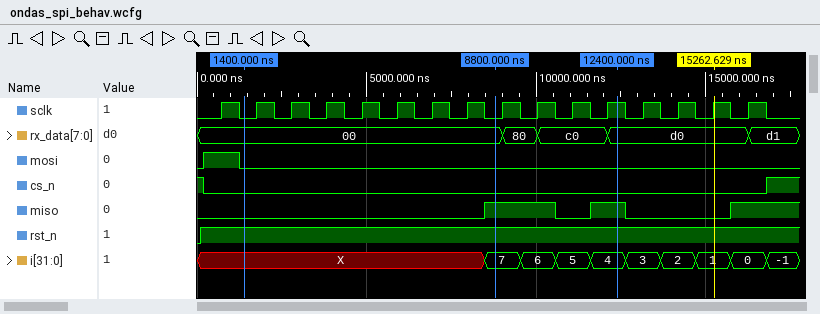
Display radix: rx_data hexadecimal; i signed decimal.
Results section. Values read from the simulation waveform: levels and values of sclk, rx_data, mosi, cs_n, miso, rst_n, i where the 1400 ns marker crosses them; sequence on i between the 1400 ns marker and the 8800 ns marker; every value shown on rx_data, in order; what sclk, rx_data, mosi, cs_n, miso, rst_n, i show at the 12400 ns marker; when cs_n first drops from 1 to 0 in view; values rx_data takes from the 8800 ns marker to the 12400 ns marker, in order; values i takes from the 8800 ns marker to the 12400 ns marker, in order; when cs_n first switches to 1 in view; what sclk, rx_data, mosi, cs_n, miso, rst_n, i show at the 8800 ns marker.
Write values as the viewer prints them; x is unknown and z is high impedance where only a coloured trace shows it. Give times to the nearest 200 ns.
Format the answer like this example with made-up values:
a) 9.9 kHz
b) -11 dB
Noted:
a) sclk=0, rx_data=00, mosi=0, cs_n=0, miso=0, rst_n=1, i=X
b) X, 7
c) 00, 80, c0, d0, d1
d) sclk=1, rx_data=d0, mosi=0, cs_n=0, miso=1, rst_n=1, i=4
e) 200 ns
f) 00, 80, c0, d0
g) 7, 6, 5, 4
h) 16800 ns
i) sclk=0, rx_data=00, mosi=0, cs_n=0, miso=1, rst_n=1, i=7
